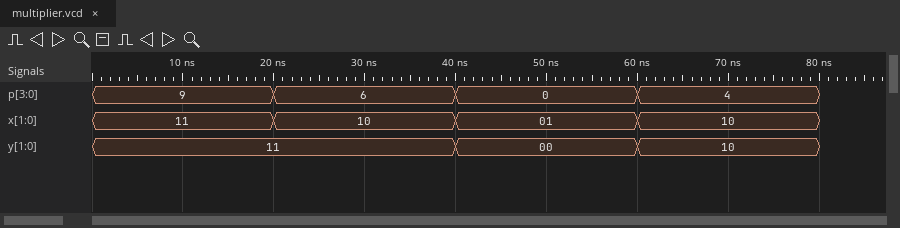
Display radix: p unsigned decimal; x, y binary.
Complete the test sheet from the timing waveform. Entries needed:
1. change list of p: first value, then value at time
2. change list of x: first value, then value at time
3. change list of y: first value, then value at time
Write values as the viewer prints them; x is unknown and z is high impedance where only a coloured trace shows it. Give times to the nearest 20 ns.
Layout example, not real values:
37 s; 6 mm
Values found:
9, 6 at 20 ns, 0 at 40 ns, 4 at 60 ns; 11, 10 at 20 ns, 01 at 40 ns, 10 at 60 ns; 11, 00 at 40 ns, 10 at 60 ns
